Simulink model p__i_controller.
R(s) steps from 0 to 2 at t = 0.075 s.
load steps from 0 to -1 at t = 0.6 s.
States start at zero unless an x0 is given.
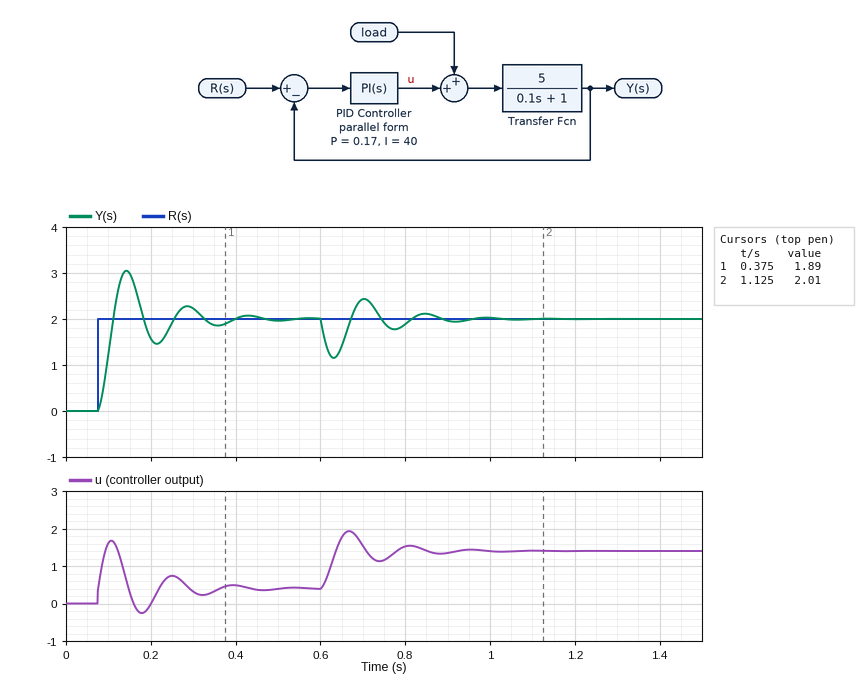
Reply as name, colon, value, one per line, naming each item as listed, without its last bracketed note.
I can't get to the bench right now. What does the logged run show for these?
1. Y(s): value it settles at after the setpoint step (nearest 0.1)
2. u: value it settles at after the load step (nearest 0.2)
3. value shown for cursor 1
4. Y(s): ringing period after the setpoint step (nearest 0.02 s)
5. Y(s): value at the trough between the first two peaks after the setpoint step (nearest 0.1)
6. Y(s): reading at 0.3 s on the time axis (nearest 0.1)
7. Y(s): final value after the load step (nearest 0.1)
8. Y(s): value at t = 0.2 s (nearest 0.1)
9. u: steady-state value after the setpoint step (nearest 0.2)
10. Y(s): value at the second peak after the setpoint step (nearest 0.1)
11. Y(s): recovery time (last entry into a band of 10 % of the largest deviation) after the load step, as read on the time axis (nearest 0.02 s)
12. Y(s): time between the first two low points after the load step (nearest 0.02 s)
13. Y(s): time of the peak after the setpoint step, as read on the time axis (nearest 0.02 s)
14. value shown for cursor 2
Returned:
Y(s): value it settles at after the setpoint step: 2.0
u: value it settles at after the load step: 1.4
value shown for cursor 1: 1.89
Y(s): ringing period after the setpoint step: 0.14 s
Y(s): value at the trough between the first two peaks after the setpoint step: 1.5
Y(s): reading at 0.3 s on the time axis: 2.2
Y(s): final value after the load step: 2.0
Y(s): value at t = 0.2 s: 1.6
u: steady-state value after the setpoint step: 0.4
Y(s): value at the second peak after the setpoint step: 2.3
Y(s): recovery time (last entry into a band of 10 % of the largest deviation) after the load step, as read on the time axis: 0.86 s
Y(s): time between the first two low points after the load step: 0.14 s
Y(s): time of the peak after the setpoint step, as read on the time axis: 0.14 s
value shown for cursor 2: 2.01
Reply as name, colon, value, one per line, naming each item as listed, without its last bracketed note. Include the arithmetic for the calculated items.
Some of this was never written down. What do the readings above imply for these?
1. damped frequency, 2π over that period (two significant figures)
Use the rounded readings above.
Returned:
damped frequency, 2π over that period: 2π / 0.14 = 45 rad/s
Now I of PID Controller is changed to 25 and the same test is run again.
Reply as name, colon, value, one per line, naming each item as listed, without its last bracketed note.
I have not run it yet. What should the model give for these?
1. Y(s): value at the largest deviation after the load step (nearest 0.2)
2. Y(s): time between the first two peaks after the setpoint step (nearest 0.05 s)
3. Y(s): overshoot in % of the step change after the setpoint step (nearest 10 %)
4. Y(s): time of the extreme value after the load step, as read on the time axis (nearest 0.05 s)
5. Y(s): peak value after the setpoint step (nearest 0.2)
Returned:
Y(s): value at the largest deviation after the load step: 1.0
Y(s): time between the first two peaks after the setpoint step: 0.20 s
Y(s): overshoot in % of the step change after the setpoint step: 40 %
Y(s): time of the extreme value after the load step, as read on the time axis: 0.65 s
Y(s): peak value after the setpoint step: 2.8
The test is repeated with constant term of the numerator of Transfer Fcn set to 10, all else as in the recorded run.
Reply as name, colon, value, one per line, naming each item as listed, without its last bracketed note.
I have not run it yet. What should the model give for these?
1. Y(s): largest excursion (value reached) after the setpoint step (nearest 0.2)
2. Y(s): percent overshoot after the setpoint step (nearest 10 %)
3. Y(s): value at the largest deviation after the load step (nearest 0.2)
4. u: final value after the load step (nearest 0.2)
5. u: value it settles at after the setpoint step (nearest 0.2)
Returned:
Y(s): largest excursion (value reached) after the setpoint step: 3.0
Y(s): percent overshoot after the setpoint step: 50 %
Y(s): value at the largest deviation after the load step: 0.8
u: final value after the load step: 1.2
u: value it settles at after the setpoint step: 0.2
